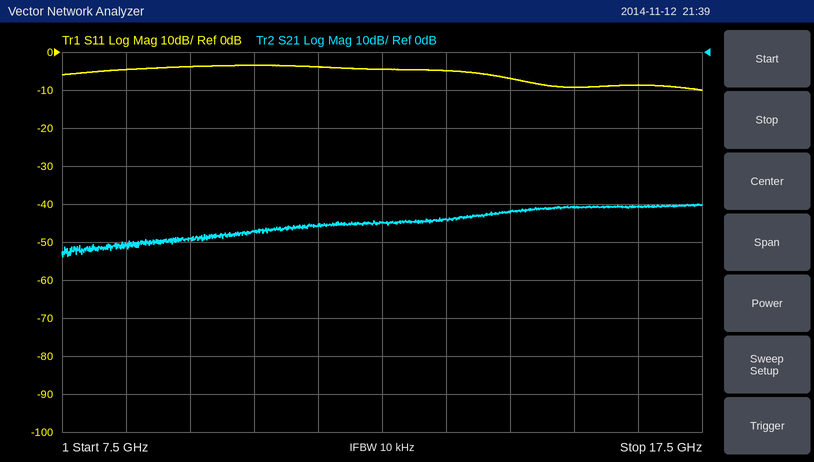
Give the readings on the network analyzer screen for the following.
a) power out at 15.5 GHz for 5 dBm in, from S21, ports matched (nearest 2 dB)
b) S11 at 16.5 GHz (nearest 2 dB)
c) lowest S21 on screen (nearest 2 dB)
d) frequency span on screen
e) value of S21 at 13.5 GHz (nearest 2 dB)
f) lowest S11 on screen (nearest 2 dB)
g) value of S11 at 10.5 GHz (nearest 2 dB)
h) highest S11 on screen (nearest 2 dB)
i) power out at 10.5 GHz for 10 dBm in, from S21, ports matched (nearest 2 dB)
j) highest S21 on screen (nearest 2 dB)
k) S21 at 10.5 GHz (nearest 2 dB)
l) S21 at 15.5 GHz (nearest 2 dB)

-36 dBm
-8 dB
-54 dB
10 GHz
-44 dB
-10 dB
-4 dB
-4 dB
-38 dBm
-40 dB
-48 dB
-40 dB
